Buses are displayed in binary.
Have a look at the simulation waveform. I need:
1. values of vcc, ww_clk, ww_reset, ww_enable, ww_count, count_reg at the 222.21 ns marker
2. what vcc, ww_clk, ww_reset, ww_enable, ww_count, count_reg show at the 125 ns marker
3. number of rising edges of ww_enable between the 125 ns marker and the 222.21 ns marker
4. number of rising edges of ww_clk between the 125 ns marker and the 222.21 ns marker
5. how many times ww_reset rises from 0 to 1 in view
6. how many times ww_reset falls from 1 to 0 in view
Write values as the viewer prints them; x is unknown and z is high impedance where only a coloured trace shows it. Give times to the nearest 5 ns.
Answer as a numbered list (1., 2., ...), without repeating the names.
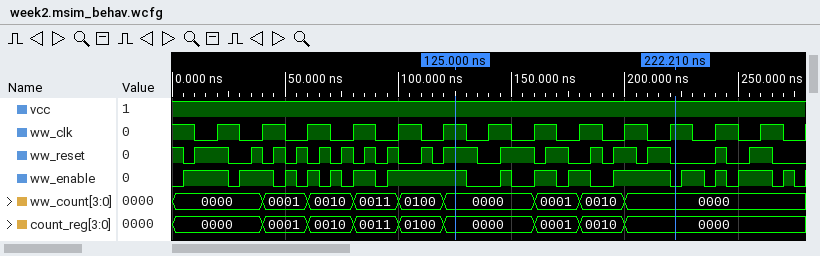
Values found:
1. vcc=1, ww_clk=1, ww_reset=0, ww_enable=0, ww_count=0000, count_reg=0000
2. vcc=1, ww_clk=1, ww_reset=1, ww_enable=1, ww_count=0000, count_reg=0000
3. 4
4. 5
5. 17
6. 18
